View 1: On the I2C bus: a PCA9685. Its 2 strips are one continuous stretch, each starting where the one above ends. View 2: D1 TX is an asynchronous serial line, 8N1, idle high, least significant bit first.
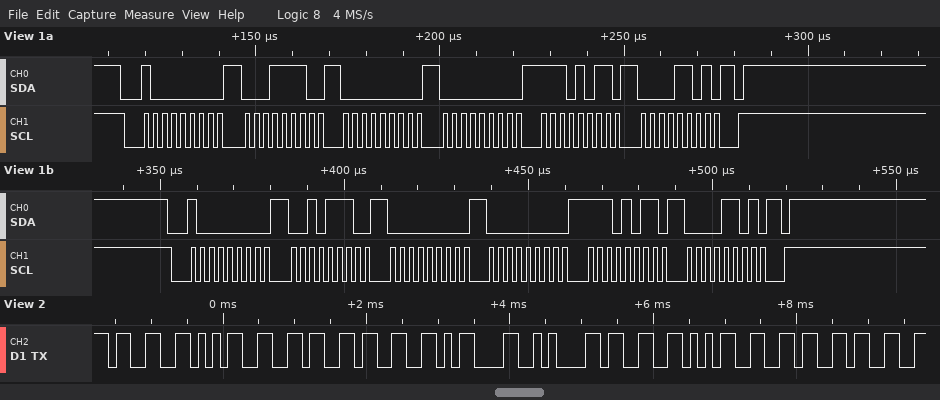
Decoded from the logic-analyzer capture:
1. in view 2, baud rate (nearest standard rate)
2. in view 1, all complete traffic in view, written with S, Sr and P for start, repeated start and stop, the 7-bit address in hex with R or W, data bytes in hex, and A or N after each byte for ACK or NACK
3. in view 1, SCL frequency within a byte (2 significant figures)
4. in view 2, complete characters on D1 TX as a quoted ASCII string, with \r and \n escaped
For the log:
9600 baud
S 40W A 1E A 00 A 00 A EB A 0D A P S 40W A 2E A 00 A 00 A EB A 0D A P
400 kHz
"3563\r\n3563"
